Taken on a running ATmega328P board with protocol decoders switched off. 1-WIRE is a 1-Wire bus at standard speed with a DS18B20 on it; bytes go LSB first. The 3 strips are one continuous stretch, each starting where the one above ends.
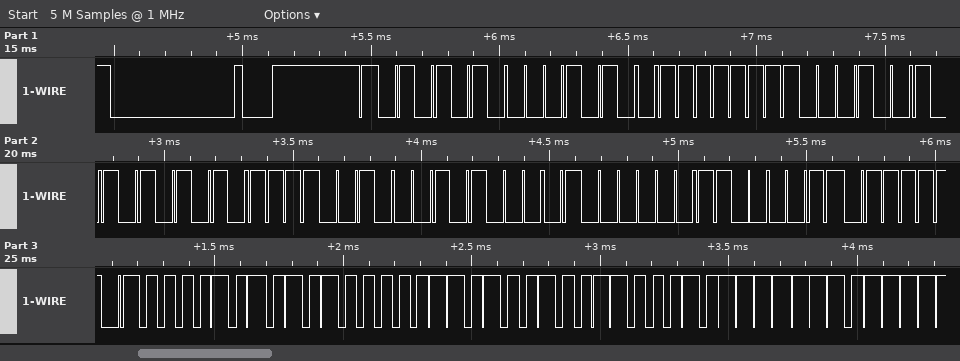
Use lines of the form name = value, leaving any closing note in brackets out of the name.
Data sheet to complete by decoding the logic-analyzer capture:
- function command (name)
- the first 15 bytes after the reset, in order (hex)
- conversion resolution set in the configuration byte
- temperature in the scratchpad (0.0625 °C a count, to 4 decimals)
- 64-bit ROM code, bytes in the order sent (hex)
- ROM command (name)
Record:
function command = Read Scratchpad
the first 15 bytes after the reset, in order = 55 28 FF 48 55 4F 14 02 C3 BE 50 05 4B 46 7F
conversion resolution set in the configuration byte = 12 bits
temperature in the scratchpad = 85.0000 °C
64-bit ROM code, bytes in the order sent = 28 FF 48 55 4F 14 02 C3
ROM command = Match ROM
